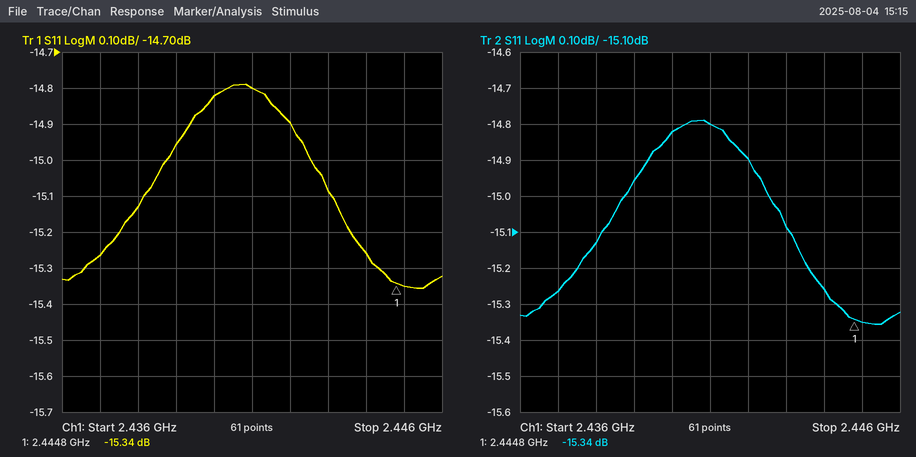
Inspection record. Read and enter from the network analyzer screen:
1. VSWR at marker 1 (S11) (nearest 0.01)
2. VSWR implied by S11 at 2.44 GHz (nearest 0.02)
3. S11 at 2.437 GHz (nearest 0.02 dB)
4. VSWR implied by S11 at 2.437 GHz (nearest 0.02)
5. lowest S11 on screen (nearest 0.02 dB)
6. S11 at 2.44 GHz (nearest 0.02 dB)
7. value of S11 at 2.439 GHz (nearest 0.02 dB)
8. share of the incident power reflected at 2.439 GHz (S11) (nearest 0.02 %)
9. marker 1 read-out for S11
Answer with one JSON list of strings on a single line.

["1.41", "1.44", "-15.26 dB", "1.42", "-15.36 dB", "-14.82 dB", "-14.96 dB", "3.20 %", "-15.34 dB"]
